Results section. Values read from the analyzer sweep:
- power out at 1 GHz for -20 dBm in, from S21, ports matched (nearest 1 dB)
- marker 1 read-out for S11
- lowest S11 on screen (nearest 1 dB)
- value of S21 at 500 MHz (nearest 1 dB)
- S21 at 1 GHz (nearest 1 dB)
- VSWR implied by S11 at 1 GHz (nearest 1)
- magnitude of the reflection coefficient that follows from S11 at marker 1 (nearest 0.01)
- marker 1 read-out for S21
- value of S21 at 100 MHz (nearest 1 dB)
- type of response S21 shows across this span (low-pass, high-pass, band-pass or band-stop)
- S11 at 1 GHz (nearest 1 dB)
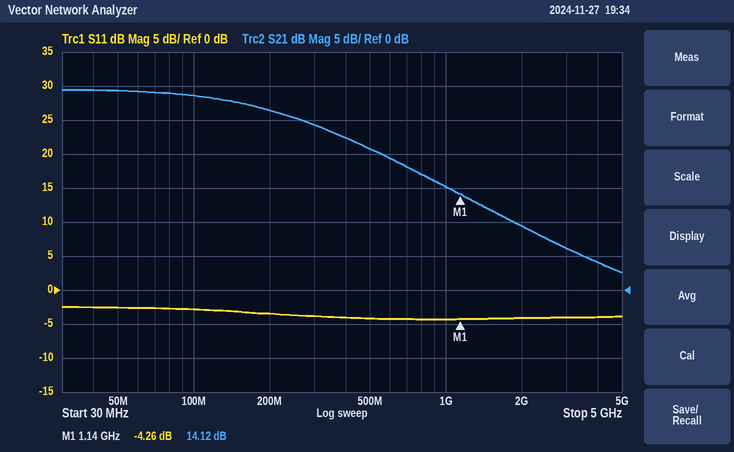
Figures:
-5 dBm
-4.26 dB
-4 dB
21 dB
15 dB
4
0.61
14.12 dB
29 dB
low-pass
-4 dB
